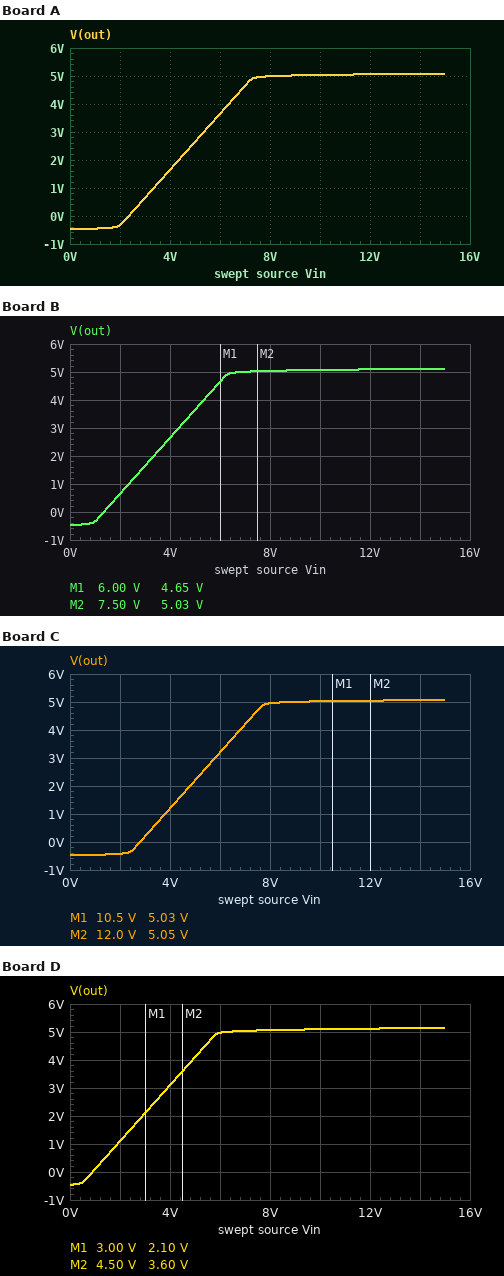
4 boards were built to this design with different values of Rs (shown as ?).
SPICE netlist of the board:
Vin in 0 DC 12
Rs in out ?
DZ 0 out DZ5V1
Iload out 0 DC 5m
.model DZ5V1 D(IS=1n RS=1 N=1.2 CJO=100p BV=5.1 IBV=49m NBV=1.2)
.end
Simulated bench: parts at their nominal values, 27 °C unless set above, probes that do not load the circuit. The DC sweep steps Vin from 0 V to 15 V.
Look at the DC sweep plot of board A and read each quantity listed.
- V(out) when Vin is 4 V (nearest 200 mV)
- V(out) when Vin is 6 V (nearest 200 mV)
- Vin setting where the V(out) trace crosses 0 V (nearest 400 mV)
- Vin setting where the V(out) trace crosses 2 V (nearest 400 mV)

1.6 V
3.6 V
2.4 V
4.4 V
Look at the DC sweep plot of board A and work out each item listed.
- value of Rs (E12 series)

470 Ω
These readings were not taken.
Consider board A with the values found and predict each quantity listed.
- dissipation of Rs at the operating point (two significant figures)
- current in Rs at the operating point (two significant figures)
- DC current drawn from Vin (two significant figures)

100 mW
15 mA
15 mA
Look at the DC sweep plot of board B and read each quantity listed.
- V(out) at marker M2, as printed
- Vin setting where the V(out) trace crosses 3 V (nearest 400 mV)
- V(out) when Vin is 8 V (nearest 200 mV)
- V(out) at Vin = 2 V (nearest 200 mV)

5.03 V
4.4 V
5.0 V
600 mV
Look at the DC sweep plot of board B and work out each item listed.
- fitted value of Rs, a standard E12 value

270 Ω
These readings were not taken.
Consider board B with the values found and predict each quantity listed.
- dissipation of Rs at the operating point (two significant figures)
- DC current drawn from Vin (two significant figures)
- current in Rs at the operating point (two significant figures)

180 mW
26 mA
26 mA
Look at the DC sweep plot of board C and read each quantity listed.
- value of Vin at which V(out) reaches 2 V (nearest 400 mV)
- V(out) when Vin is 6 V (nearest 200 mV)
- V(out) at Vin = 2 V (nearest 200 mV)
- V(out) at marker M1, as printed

4.8 V
3.2 V
-400 mV
5.03 V
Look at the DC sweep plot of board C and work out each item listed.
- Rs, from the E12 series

560 Ω
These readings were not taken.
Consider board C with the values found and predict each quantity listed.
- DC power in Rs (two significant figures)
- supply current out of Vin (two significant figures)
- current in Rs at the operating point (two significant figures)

86 mW
12 mA
12 mA
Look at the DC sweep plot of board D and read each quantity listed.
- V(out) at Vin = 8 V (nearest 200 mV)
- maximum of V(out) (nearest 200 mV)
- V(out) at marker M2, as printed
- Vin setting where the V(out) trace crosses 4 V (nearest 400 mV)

5.0 V
5.2 V
3.60 V
4.8 V
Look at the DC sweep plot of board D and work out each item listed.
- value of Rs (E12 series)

180 Ω
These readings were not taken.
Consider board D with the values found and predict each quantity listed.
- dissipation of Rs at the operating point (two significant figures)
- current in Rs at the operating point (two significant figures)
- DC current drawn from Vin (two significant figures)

260 mW
38 mA
38 mA
